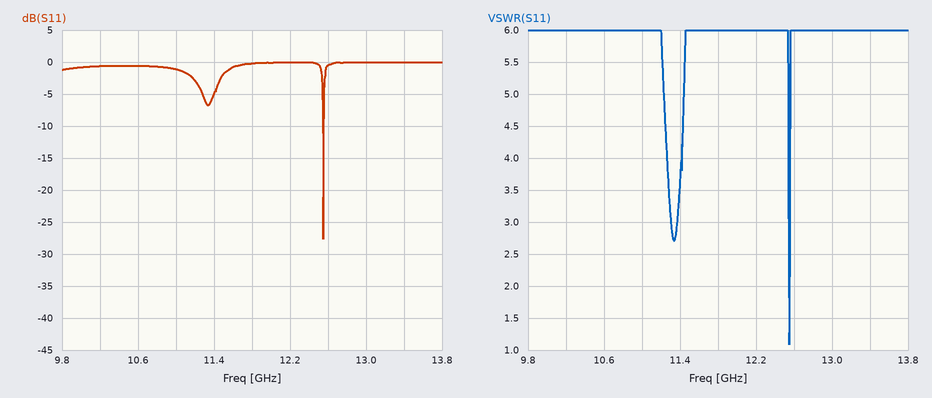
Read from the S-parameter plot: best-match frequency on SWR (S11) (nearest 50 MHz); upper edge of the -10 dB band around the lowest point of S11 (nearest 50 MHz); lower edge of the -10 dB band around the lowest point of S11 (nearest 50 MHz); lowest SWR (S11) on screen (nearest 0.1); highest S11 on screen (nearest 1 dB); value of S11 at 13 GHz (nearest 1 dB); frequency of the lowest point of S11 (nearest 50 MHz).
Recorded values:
12.55 GHz
12.55 GHz
12.55 GHz
1.1
0 dB
0 dB
12.55 GHz
